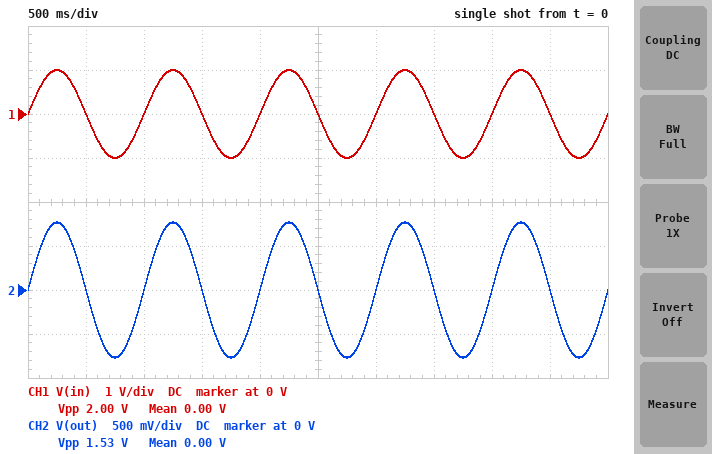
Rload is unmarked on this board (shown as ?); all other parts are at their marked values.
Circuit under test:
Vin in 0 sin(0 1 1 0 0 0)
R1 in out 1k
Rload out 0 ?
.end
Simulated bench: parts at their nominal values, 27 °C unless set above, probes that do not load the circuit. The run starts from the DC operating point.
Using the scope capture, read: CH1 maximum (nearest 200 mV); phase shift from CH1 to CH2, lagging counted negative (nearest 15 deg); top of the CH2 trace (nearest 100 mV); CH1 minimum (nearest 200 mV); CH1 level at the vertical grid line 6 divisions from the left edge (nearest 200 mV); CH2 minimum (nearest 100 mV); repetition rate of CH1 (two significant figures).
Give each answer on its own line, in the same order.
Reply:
1.0 V
0 deg
800 mV
-1.0 V
0 V
-800 mV
1.0 Hz
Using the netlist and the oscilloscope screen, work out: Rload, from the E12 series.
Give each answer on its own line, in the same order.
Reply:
3.3 kΩ
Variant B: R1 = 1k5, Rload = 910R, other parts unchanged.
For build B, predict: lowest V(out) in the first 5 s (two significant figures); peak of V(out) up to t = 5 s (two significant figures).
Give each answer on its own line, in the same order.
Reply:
-380 mV
380 mV
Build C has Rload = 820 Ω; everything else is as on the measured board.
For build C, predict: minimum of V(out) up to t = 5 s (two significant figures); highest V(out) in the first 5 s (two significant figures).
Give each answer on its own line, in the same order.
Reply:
-450 mV
450 mV
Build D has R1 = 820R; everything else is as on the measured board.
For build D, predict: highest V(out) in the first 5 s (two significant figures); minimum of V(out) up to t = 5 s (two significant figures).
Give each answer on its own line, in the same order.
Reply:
800 mV
-800 mV
